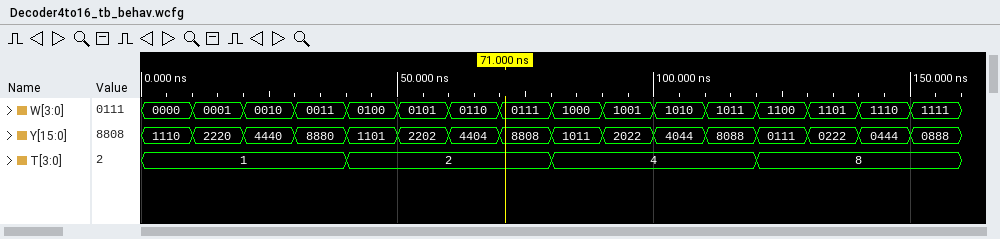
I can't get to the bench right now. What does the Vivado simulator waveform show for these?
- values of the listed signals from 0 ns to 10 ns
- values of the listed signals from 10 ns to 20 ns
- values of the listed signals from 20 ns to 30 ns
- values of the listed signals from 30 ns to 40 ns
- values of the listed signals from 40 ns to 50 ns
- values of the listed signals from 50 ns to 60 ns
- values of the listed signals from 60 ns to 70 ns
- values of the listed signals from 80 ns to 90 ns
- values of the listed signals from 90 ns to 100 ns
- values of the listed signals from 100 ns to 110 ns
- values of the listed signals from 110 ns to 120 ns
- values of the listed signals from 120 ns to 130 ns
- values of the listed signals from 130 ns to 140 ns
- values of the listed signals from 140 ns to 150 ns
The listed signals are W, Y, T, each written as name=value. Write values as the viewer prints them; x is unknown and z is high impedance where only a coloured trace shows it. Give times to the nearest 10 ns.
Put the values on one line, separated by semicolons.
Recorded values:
W=0000, Y=1110, T=1; W=0001, Y=2220, T=1; W=0010, Y=4440, T=1; W=0011, Y=8880, T=1; W=0100, Y=1101, T=2; W=0101, Y=2202, T=2; W=0110, Y=4404, T=2; W=1000, Y=1011, T=4; W=1001, Y=2022, T=4; W=1010, Y=4044, T=4; W=1011, Y=8088, T=4; W=1100, Y=0111, T=8; W=1101, Y=0222, T=8; W=1110, Y=0444, T=8
